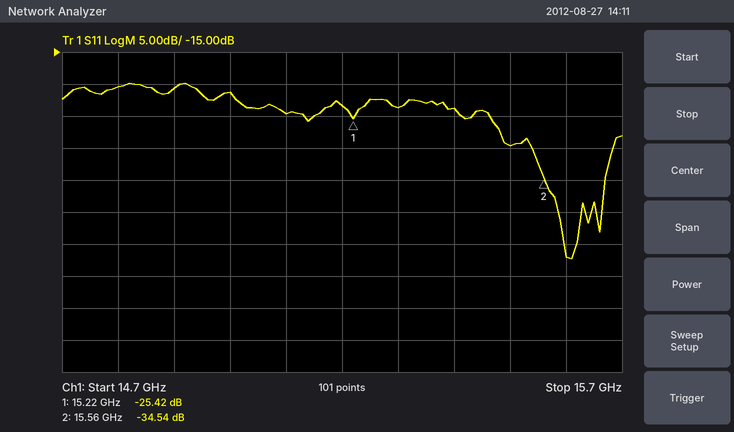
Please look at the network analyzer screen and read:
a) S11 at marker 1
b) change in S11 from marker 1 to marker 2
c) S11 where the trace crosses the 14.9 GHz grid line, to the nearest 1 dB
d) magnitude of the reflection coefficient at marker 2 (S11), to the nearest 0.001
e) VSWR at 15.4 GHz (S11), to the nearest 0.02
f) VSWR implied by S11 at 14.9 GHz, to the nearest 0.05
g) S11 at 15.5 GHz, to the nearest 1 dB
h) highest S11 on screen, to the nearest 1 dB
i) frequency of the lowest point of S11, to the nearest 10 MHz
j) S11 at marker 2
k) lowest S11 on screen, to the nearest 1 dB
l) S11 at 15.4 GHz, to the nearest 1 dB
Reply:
-25.42 dB
-9.12 dB
-21 dB
0.019
1.14
1.20
-30 dB
-20 dB
15.61 GHz
-34.54 dB
-47 dB
-24 dB
